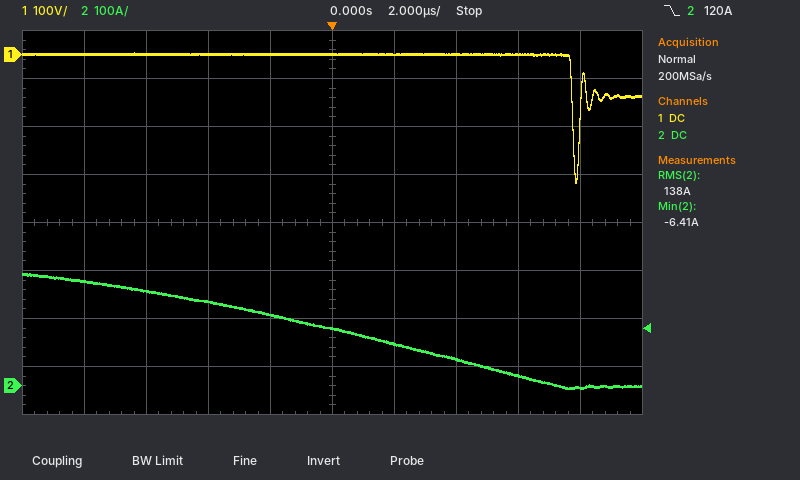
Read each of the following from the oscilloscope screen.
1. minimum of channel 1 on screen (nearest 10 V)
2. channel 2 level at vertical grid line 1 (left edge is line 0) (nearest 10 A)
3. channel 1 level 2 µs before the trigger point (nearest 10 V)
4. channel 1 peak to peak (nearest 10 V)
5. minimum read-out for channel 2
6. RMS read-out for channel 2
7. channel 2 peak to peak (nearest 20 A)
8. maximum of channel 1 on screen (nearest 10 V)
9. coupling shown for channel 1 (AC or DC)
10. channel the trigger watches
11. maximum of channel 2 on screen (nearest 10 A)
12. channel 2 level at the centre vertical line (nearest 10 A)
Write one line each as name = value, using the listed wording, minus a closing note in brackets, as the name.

minimum of channel 1 on screen = -270 V
channel 2 level at vertical grid line 1 (left edge is line 0) = 220 A
channel 1 level 2 µs before the trigger point = 0 V
channel 1 peak to peak = 270 V
minimum read-out for channel 2 = -6.41 A
RMS read-out for channel 2 = 138 A
channel 2 peak to peak = 240 A
maximum of channel 1 on screen = 0 V
coupling shown for channel 1 = DC
channel the trigger watches = channel 2
maximum of channel 2 on screen = 230 A
channel 2 level at the centre vertical line = 120 A
